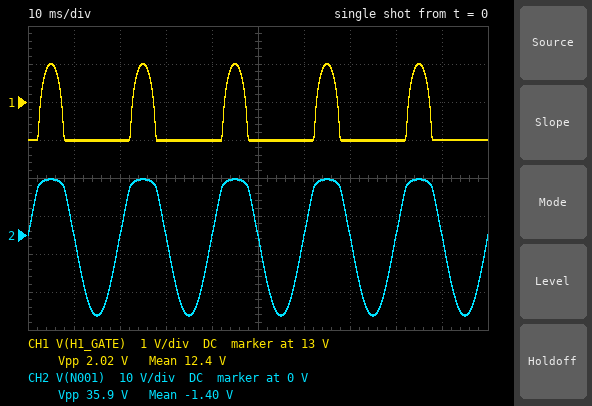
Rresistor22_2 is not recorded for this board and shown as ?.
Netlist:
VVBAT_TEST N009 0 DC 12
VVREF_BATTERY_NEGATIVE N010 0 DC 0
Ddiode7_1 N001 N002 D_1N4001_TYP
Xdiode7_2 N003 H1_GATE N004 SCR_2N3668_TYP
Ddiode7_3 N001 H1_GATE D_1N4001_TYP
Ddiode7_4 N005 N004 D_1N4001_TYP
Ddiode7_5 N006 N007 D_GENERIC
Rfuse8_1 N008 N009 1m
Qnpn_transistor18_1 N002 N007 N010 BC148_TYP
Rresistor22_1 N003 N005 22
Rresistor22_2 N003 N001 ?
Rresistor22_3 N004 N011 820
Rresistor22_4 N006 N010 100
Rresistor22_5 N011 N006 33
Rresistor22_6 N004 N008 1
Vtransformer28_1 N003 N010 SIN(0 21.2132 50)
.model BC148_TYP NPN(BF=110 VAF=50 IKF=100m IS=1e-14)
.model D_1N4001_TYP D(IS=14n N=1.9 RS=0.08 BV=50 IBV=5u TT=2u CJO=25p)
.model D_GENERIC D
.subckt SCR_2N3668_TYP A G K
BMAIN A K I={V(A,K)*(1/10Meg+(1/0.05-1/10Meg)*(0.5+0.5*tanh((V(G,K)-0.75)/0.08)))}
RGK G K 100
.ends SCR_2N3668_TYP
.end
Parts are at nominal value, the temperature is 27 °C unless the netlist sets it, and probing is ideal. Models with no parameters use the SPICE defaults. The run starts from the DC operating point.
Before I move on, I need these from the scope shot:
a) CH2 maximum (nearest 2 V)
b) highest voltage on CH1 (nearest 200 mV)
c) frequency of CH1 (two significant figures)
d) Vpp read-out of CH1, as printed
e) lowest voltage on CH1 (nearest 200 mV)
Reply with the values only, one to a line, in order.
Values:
14 V
14.0 V
50 Hz
2.02 V
12.0 V
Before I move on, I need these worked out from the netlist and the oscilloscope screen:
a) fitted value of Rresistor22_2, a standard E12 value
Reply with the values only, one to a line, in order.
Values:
150 Ω
